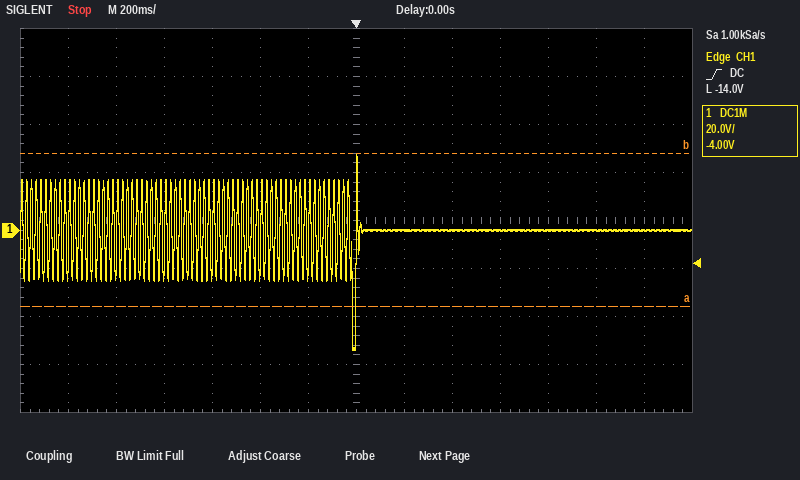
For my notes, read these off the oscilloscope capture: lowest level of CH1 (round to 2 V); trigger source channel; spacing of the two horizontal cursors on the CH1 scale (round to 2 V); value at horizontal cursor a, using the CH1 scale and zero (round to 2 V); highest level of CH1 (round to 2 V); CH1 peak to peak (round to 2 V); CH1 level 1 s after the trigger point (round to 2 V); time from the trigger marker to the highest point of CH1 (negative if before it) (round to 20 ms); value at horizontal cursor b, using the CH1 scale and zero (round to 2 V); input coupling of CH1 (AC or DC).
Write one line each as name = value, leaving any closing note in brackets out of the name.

lowest level of CH1 = -50 V
trigger source channel = CH1
spacing of the two horizontal cursors on the CH1 scale = 64 V
value at horizontal cursor a, using the CH1 scale and zero = -32 V
highest level of CH1 = 32 V
CH1 peak to peak = 82 V
CH1 level 1 s after the trigger point = 0 V
time from the trigger marker to the highest point of CH1 (negative if before it) = 0 ms
value at horizontal cursor b, using the CH1 scale and zero = 32 V
input coupling of CH1 = DC
